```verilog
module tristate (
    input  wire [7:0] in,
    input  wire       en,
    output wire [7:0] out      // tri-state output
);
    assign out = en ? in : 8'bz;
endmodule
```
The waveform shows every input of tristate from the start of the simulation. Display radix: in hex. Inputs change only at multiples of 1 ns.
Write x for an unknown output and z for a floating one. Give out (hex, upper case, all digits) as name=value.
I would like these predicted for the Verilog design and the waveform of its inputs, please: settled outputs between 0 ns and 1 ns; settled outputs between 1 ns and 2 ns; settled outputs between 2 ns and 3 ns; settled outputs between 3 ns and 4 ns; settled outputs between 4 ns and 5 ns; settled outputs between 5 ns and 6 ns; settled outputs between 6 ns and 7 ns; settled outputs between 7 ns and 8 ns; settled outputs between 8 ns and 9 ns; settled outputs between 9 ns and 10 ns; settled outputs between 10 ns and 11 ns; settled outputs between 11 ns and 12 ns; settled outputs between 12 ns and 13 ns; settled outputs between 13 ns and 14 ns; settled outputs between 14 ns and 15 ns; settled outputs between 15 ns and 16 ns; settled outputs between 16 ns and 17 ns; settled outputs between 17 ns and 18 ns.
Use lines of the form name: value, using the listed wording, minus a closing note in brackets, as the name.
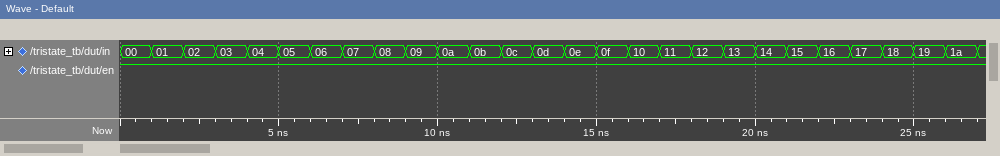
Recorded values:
settled outputs between 0 ns and 1 ns: out=00
settled outputs between 1 ns and 2 ns: out=01
settled outputs between 2 ns and 3 ns: out=02
settled outputs between 3 ns and 4 ns: out=03
settled outputs between 4 ns and 5 ns: out=04
settled outputs between 5 ns and 6 ns: out=05
settled outputs between 6 ns and 7 ns: out=06
settled outputs between 7 ns and 8 ns: out=07
settled outputs between 8 ns and 9 ns: out=08
settled outputs between 9 ns and 10 ns: out=09
settled outputs between 10 ns and 11 ns: out=0A
settled outputs between 11 ns and 12 ns: out=0B
settled outputs between 12 ns and 13 ns: out=0C
settled outputs between 13 ns and 14 ns: out=0D
settled outputs between 14 ns and 15 ns: out=0E
settled outputs between 15 ns and 16 ns: out=0F
settled outputs between 16 ns and 17 ns: out=10
settled outputs between 17 ns and 18 ns: out=11
